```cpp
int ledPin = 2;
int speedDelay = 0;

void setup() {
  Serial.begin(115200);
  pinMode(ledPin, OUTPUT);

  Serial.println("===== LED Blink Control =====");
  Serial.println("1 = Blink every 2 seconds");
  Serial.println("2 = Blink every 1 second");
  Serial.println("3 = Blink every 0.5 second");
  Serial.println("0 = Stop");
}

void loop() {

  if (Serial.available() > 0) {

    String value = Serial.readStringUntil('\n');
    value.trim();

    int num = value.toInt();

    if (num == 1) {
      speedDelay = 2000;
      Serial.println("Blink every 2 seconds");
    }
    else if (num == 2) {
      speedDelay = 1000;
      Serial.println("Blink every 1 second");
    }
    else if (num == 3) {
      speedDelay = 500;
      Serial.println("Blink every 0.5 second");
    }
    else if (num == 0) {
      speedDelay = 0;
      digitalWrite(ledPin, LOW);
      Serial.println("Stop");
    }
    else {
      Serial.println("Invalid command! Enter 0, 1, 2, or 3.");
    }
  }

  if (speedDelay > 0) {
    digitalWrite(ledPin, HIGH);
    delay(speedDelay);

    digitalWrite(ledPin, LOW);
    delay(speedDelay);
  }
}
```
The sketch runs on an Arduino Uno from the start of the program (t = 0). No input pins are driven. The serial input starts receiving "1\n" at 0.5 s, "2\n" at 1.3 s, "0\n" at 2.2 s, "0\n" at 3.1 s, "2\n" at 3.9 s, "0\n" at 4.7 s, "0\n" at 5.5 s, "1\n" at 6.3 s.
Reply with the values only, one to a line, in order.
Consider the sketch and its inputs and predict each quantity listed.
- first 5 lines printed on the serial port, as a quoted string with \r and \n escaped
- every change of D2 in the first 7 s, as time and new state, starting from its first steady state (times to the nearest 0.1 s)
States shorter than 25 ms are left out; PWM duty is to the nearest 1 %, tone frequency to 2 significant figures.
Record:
"===== LED Blink Control =====\r\n1 = Blink every 2 seconds\r\n2 = Blink every 1 second\r\n3 = Blink every 0.5 second\r\n0 = Stop\r\n"
0 s low; 0.5 s high; 2.5 s low; 4.5 s high; 5.5 s low; 6.5 s high
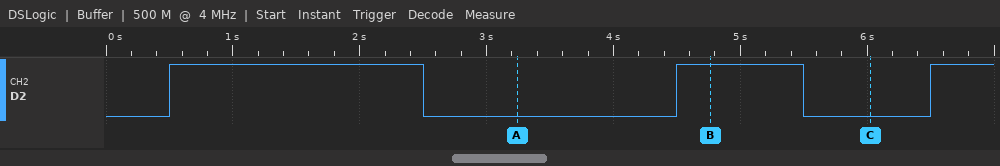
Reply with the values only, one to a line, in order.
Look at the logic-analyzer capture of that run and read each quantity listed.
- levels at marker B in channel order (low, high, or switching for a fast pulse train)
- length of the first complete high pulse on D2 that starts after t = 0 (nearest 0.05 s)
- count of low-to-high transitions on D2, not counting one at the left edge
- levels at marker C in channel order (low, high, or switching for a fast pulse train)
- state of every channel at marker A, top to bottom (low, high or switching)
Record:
D2 high
2.00 s
3
D2 low
D2 low
